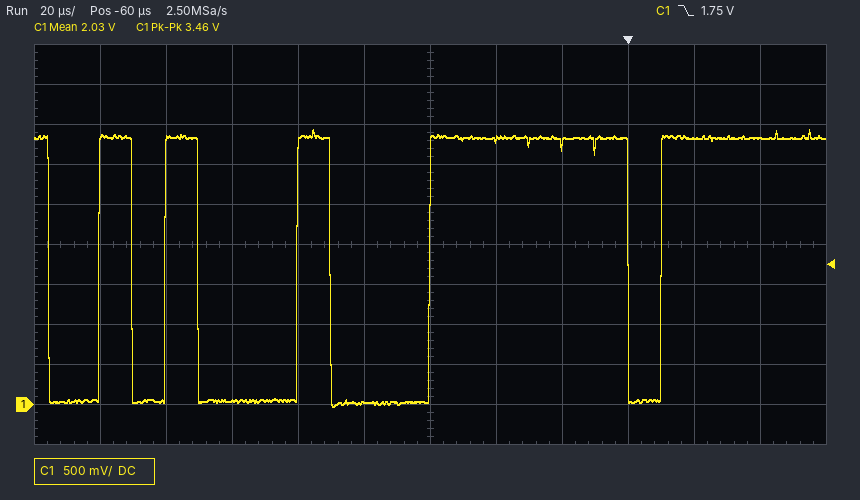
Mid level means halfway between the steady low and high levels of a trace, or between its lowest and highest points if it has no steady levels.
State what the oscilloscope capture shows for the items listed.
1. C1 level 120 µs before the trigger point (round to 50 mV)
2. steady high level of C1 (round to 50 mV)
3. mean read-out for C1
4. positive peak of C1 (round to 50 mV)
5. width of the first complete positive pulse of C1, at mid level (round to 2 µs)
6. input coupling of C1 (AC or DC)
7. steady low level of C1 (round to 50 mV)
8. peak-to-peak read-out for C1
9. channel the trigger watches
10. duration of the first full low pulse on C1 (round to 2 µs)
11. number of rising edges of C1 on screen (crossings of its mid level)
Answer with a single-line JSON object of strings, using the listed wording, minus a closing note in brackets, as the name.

{"C1 level 120 µs before the trigger point": "50 mV", "steady high level of C1": "3.35 V", "mean read-out for C1": "2.03 V", "positive peak of C1": "3.45 V", "width of the first complete positive pulse of C1, at mid level": "10 µs", "input coupling of C1": "DC", "steady low level of C1": "50 mV", "peak-to-peak read-out for C1": "3.46 V", "channel the trigger watches": "C1", "duration of the first full low pulse on C1": "16 µs", "number of rising edges of C1 on screen": "5"}
